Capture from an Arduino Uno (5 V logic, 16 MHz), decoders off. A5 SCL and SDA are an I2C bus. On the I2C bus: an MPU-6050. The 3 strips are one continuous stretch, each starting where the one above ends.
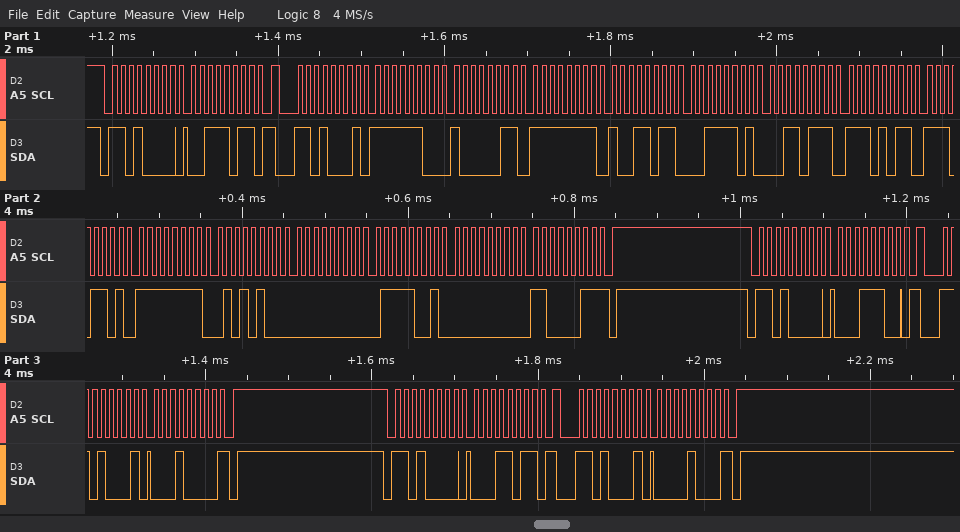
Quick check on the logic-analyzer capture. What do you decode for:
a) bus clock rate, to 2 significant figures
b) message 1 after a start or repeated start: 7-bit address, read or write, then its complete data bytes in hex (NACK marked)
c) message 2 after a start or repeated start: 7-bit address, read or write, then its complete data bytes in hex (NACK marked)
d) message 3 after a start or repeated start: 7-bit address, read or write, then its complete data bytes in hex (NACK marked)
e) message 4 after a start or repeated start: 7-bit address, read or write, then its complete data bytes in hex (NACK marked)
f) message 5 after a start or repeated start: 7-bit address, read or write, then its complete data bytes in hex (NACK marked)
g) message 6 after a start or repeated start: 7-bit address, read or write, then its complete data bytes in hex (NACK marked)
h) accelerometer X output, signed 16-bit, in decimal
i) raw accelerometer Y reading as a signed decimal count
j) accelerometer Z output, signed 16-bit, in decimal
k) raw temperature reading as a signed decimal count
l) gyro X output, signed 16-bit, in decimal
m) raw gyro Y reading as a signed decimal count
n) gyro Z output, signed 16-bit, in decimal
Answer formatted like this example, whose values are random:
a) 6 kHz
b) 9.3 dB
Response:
a) 100 kHz
b) 0x68 write: 3B
c) 0x68 read: FC 83 FF 9B 3D 37 EB ED FF 54 00 79 00 C3 NACK
d) 0x68 write: 1C
e) 0x68 read: 10 NACK
f) 0x68 write: 1B
g) 0x68 read: 08 NACK
h) -893
i) -101
j) 15671
k) -5139
l) -172
m) 121
n) 195
